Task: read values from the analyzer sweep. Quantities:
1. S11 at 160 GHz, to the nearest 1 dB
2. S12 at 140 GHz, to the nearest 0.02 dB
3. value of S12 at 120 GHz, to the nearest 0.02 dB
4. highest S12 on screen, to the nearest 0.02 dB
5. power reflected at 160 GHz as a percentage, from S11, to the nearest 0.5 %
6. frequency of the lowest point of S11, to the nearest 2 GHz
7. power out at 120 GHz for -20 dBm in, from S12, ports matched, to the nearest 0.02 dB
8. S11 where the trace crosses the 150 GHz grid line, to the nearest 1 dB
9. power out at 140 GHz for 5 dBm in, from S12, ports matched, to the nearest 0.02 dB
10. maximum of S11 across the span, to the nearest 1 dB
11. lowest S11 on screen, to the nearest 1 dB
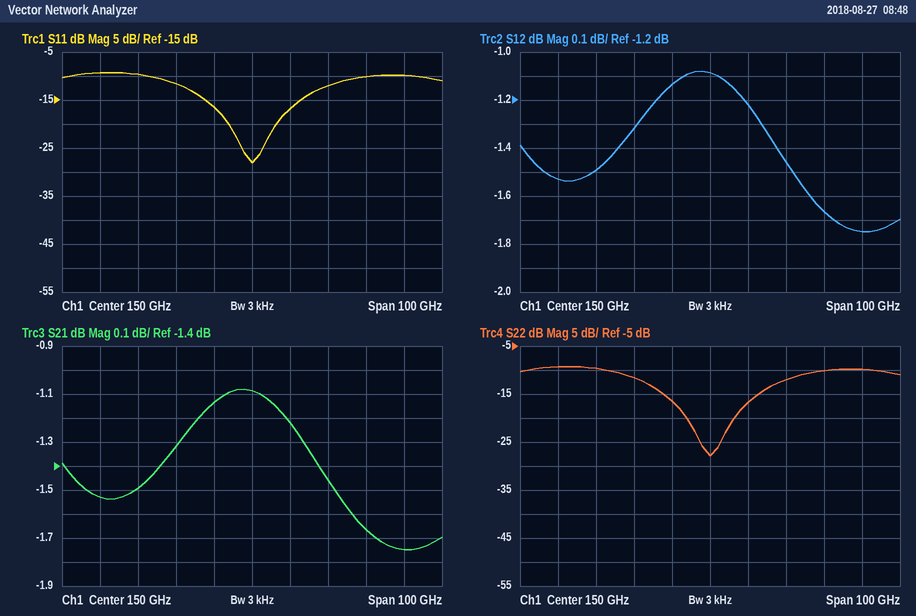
-17 dB
-1.14 dB
-1.50 dB
-1.08 dB
2.0 %
150 GHz
-21.50 dBm
-28 dB
3.86 dBm
-9 dB
-28 dB
